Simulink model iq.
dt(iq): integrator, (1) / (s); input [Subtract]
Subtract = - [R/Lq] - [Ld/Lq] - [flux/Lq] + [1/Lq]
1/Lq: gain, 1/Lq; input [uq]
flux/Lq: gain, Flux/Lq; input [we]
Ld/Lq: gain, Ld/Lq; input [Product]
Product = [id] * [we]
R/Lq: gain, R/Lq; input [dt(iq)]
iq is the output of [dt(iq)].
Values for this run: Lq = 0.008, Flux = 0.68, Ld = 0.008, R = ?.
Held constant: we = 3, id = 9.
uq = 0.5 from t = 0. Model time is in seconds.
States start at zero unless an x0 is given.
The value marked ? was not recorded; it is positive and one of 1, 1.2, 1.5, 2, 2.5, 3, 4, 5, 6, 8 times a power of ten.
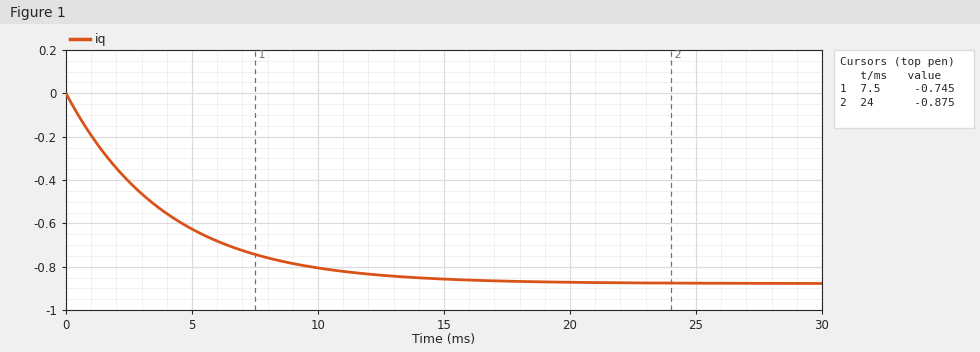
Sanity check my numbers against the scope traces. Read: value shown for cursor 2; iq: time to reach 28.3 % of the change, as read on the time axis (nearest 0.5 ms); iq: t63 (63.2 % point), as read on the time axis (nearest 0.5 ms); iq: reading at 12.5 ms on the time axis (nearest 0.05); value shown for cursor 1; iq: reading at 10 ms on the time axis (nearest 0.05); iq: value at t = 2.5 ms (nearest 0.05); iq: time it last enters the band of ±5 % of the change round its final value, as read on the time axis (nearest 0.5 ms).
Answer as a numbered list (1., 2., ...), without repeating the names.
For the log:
1. -0.875
2. 1.5 ms
3. 4.0 ms
4. -0.85
5. -0.745
6. -0.80
7. -0.40
8. 12.0 ms
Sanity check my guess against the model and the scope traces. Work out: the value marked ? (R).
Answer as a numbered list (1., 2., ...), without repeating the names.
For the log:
1. 2
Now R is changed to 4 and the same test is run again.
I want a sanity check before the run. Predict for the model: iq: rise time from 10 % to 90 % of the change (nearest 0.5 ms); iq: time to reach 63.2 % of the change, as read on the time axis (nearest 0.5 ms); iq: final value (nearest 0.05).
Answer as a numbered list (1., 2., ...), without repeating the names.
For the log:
1. 4.5 ms
2. 2.0 ms
3. -0.45
